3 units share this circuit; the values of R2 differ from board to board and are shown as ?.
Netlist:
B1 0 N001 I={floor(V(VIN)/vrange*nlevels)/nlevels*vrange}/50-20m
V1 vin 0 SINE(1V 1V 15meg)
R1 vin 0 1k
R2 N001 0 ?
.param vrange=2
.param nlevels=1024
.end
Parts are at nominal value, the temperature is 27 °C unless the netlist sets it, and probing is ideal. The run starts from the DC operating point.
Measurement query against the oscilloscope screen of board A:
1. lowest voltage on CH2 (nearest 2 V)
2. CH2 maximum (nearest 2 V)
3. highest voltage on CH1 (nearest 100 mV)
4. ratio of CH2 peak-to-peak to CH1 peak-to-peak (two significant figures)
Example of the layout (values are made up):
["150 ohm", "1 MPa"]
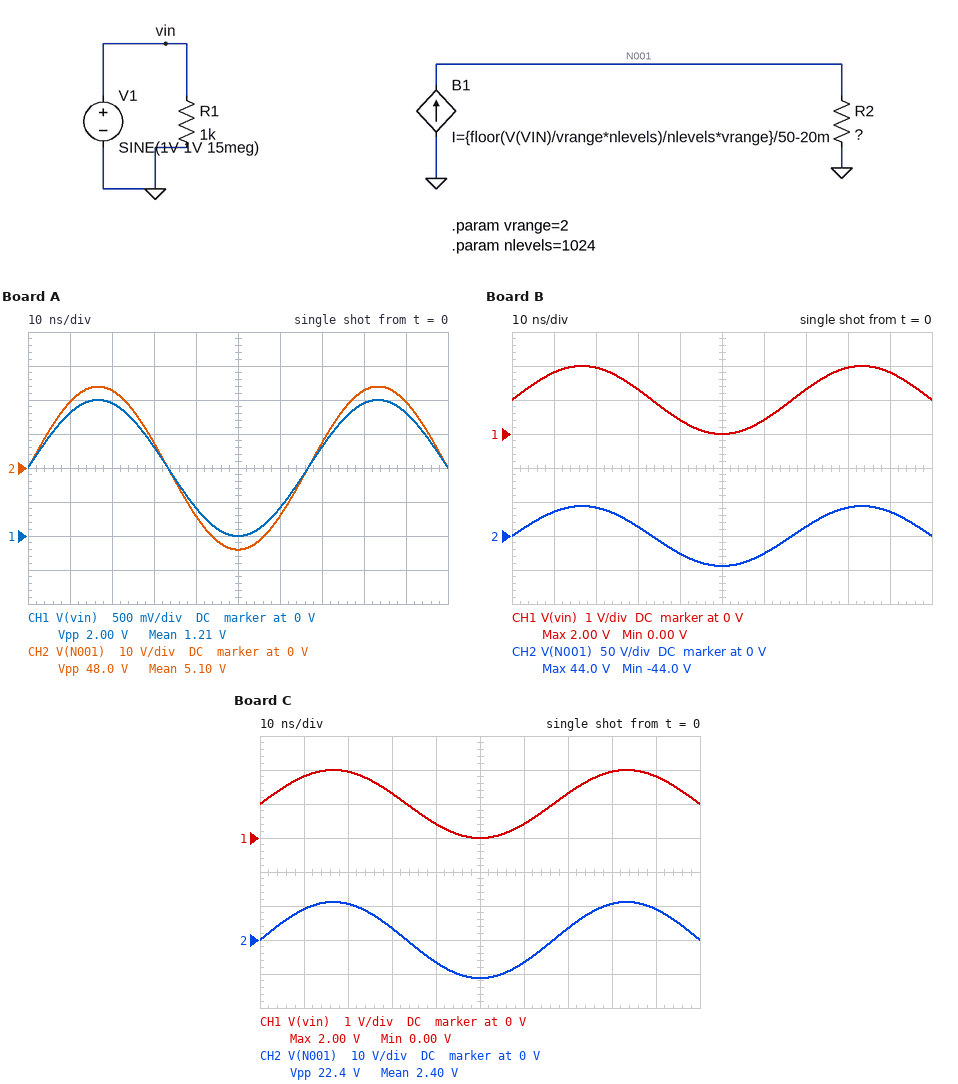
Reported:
["-24 V", "24 V", "2.0 V", "24"]
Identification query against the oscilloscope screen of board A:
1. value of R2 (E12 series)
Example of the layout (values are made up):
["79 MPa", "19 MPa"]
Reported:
["1.2 kΩ"]
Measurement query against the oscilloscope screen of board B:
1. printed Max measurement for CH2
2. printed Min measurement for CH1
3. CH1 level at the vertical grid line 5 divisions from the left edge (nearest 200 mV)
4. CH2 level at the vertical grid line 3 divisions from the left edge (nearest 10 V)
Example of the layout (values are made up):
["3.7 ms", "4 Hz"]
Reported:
["44.0 V", "0.00 V", "0 V", "10 V"]
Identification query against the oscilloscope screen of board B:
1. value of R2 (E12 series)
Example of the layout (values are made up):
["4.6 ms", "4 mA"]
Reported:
["2.2 kΩ"]
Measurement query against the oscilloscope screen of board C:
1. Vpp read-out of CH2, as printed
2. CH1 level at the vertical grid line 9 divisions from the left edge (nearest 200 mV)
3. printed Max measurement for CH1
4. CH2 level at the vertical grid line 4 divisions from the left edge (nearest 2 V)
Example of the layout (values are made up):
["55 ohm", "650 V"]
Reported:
["22.4 V", "1.8 V", "2.00 V", "-6 V"]
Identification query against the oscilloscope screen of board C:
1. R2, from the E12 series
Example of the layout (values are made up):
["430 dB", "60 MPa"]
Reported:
["560 Ω"]
